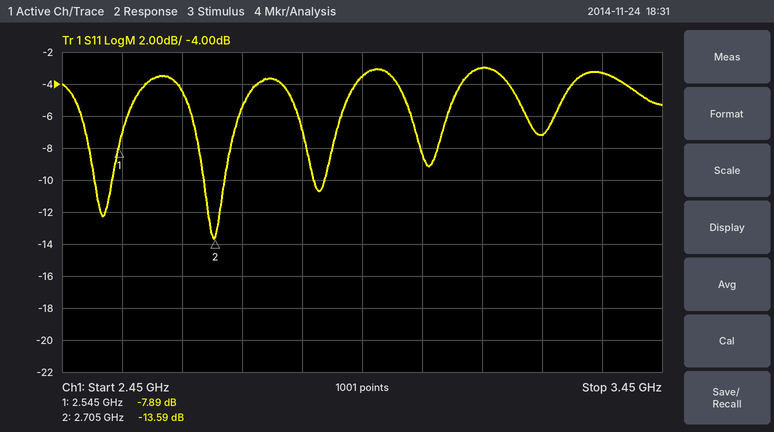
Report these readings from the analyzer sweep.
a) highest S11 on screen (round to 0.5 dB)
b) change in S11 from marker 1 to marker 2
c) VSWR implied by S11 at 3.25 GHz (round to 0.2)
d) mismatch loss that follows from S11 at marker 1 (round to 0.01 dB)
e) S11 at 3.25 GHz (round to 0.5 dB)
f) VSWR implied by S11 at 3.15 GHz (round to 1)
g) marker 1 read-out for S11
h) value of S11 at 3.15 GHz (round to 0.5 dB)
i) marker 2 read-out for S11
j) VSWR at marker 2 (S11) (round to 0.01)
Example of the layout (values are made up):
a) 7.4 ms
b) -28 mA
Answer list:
a) -3.0 dB
b) -5.70 dB
c) 2.6
d) 0.77 dB
e) -7.0 dB
f) 6
g) -7.89 dB
h) -3.0 dB
i) -13.59 dB
j) 1.53
